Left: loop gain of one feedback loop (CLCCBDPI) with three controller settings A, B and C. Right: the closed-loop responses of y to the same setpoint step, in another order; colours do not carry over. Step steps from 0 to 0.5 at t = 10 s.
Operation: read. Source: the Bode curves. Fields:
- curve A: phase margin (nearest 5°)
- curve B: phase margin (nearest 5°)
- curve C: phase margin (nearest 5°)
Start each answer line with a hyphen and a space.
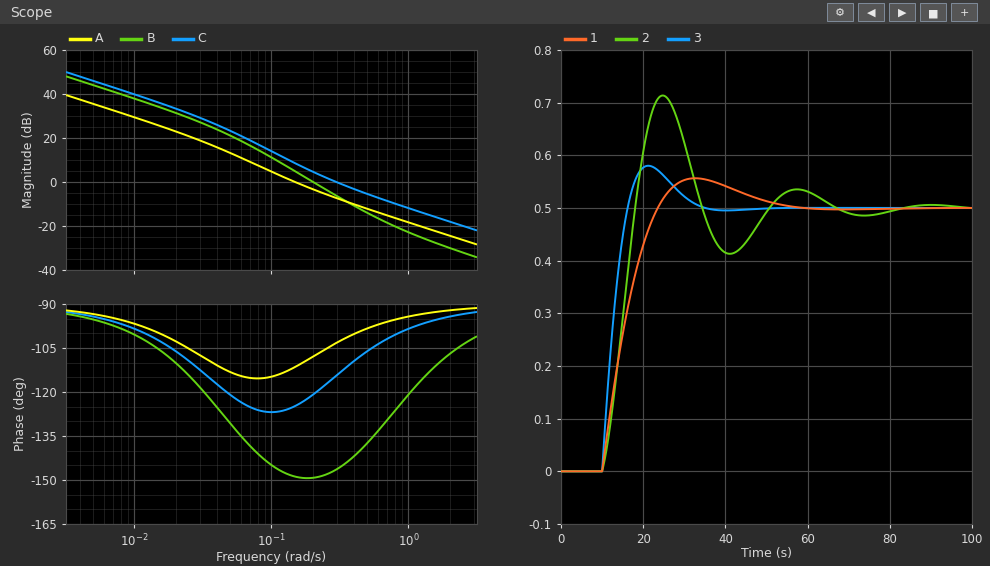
- 70°
- 30°
- 65°
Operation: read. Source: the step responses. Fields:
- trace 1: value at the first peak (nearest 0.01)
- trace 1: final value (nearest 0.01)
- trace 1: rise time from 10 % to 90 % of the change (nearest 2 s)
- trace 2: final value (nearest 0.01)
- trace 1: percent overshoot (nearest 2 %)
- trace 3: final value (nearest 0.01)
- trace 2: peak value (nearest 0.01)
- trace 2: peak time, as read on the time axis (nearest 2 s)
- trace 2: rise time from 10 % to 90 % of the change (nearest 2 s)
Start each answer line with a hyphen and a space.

- 0.56
- 0.50
- 10 s
- 0.50
- 12 %
- 0.50
- 0.71
- 24 s
- 6 s
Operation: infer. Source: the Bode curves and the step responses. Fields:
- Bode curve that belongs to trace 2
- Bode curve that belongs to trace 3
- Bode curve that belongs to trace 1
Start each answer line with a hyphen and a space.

- B
- C
- A
